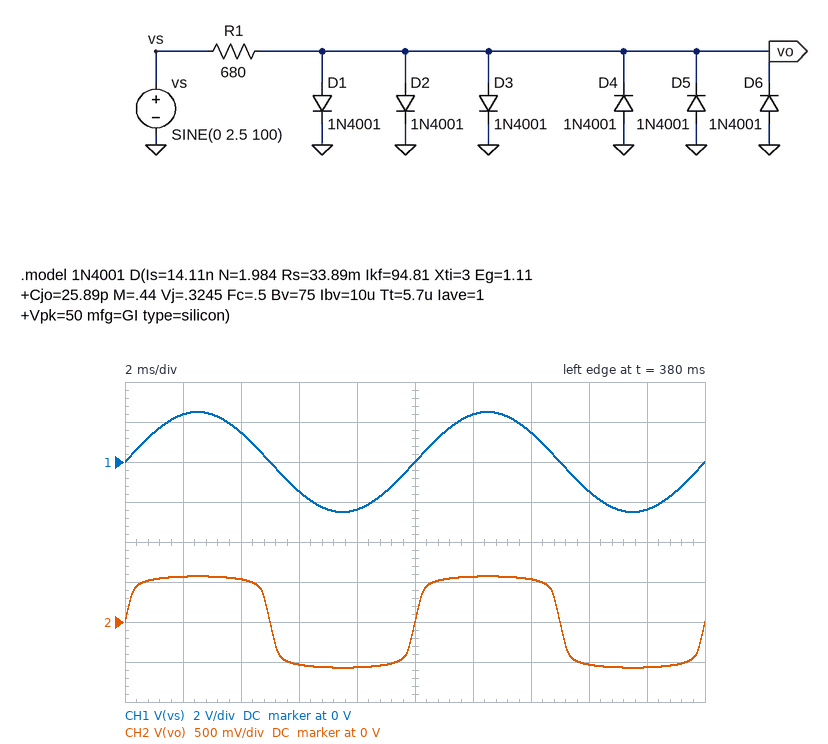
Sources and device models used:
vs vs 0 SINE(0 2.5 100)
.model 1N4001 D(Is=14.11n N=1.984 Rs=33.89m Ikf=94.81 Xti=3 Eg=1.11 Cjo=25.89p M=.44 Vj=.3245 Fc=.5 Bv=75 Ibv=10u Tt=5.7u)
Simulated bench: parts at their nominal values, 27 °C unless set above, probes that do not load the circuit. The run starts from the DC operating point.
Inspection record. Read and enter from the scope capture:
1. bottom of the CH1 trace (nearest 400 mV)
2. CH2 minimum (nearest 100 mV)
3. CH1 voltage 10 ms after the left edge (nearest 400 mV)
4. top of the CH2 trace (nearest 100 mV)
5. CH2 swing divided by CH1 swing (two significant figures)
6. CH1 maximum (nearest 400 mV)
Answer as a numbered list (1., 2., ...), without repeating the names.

1. -2.4 V
2. -600 mV
3. 0 V
4. 600 mV
5. 0.23
6. 2.4 V
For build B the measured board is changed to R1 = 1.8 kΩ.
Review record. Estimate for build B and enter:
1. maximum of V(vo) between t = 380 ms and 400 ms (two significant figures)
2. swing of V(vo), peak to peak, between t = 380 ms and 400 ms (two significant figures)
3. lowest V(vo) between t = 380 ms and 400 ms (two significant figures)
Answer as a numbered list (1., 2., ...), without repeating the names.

1. 520 mV
2. 1.0 V
3. -520 mV
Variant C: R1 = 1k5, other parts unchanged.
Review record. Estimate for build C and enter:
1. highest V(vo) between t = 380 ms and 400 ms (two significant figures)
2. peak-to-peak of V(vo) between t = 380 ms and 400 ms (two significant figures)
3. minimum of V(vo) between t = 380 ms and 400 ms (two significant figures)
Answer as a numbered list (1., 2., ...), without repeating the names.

1. 530 mV
2. 1.1 V
3. -530 mV
